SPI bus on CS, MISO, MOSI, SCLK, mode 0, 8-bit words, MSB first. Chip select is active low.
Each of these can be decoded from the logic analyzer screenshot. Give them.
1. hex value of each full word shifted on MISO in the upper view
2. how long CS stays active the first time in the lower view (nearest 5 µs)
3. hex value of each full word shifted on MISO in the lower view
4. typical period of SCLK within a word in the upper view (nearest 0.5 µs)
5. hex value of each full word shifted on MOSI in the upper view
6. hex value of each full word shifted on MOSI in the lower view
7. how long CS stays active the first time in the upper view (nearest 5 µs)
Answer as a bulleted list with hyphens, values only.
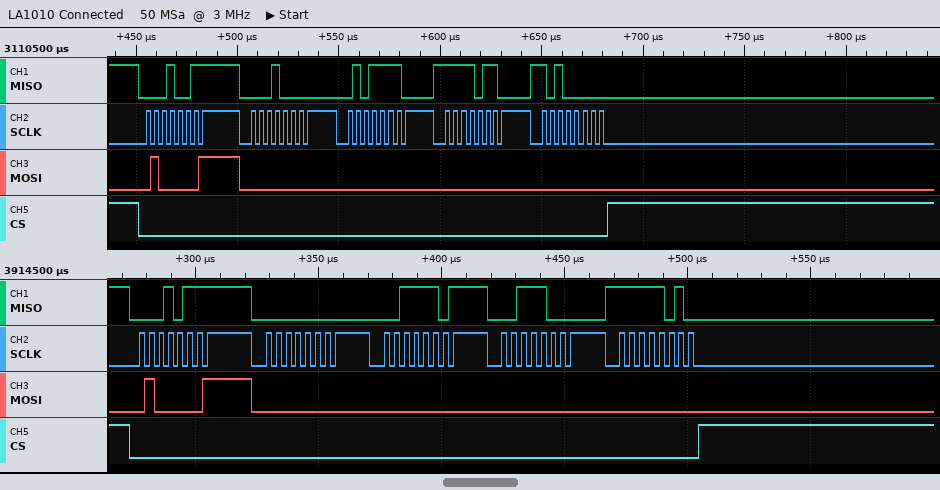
- 13, 10, 5E, F6, A0
- 230 µs
- 17, 00, 3D, 38, FA
- 4 µs
- 41, 00, 00, 00, 00
- 41, 00, 00, 00, 00
- 230 µs
